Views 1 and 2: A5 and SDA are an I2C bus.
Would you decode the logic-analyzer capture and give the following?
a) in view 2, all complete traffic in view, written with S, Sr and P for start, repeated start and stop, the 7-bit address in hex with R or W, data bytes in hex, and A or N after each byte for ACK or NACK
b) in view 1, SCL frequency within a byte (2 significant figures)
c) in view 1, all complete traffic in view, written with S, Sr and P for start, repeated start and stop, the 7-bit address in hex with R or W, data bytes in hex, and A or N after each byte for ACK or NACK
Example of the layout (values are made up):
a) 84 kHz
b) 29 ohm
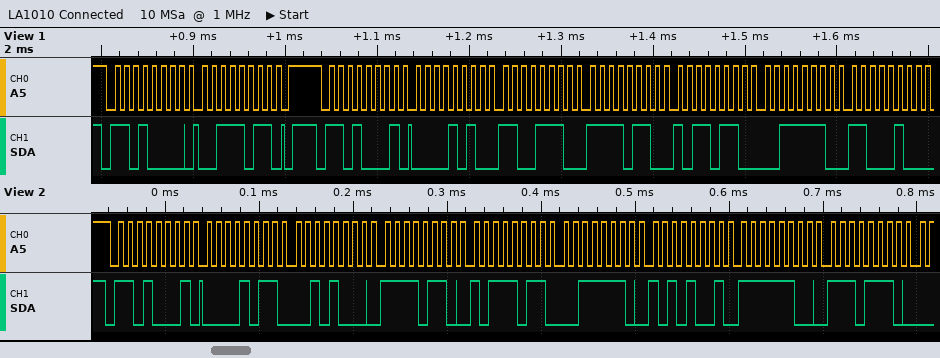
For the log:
a) S 68R A 0B A 28 A F6 A BB A 3E A A9 A FC A EE A
b) 100 kHz
c) S 68W A 3B A P S 68R A 0A A CE A F6 A B6 A 3E A C4 A
